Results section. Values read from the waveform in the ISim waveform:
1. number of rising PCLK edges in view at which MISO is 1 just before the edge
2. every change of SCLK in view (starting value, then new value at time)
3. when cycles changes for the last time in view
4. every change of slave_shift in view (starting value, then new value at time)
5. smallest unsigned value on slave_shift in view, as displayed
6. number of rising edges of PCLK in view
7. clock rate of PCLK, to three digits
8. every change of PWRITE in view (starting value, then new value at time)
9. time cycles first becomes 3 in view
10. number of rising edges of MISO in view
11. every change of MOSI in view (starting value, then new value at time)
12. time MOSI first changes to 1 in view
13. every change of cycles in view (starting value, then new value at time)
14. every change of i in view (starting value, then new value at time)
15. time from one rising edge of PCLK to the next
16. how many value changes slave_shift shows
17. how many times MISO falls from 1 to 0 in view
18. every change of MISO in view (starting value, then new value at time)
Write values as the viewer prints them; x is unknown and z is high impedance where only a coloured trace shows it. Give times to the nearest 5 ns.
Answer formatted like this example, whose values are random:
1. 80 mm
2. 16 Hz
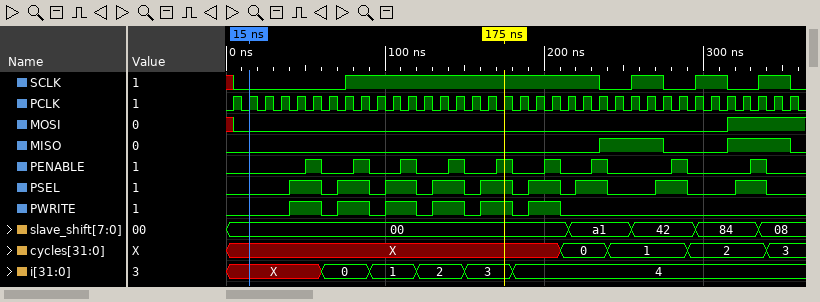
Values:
1. 8
2. x, 0 at 5 ns, 1 at 75 ns, 0 at 235 ns, 1 at 255 ns, 0 at 275 ns, 1 at 295 ns, 0 at 315 ns, 1 at 335 ns, 0 at 355 ns
3. 340 ns
4. 00, a1 at 215 ns, 42 at 255 ns, 84 at 295 ns, 08 at 335 ns
5. 00
6. 36
7. 100 MHz
8. 0, 1 at 40 ns, 0 at 60 ns, 1 at 70 ns, 0 at 90 ns, 1 at 100 ns, 0 at 120 ns, 1 at 130 ns, 0 at 150 ns, 1 at 160 ns, 0 at 180 ns, 1 at 190 ns, 0 at 210 ns
9. 340 ns
10. 2
11. x, 0 at 5 ns, 1 at 315 ns
12. 315 ns
13. X, 0 at 210 ns, 1 at 240 ns, 2 at 290 ns, 3 at 340 ns
14. X, 0 at 60 ns, 1 at 90 ns, 2 at 120 ns, 3 at 150 ns, 4 at 180 ns
15. 10 ns
16. 4
17. 2
18. 0, 1 at 235 ns, 0 at 275 ns, 1 at 315 ns, 0 at 355 ns
